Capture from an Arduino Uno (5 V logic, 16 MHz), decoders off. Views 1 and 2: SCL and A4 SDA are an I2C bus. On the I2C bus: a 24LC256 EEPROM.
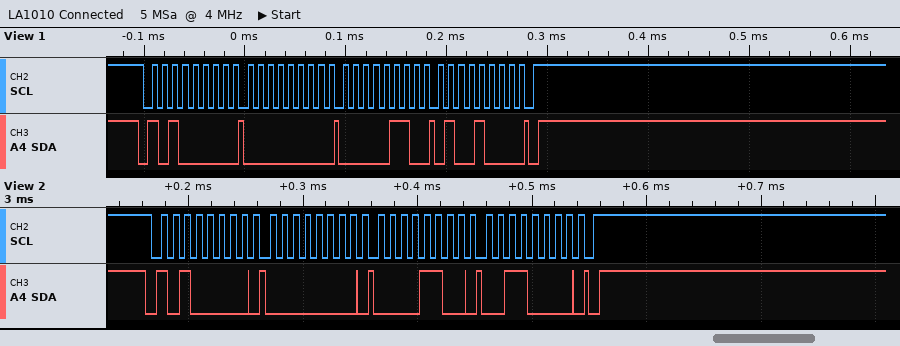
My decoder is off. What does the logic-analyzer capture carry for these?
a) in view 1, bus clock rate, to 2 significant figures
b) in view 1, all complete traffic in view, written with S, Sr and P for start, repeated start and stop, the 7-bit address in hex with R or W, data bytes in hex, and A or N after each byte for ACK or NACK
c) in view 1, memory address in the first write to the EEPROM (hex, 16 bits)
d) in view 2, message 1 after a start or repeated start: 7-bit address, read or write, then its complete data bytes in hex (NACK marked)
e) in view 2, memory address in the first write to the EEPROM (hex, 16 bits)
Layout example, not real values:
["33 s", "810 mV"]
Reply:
["100 kHz", "S 50W A 00 A 06 A 48 A P", "0x0006", "0x50 write: 00 0C 30", "0x000C"]
